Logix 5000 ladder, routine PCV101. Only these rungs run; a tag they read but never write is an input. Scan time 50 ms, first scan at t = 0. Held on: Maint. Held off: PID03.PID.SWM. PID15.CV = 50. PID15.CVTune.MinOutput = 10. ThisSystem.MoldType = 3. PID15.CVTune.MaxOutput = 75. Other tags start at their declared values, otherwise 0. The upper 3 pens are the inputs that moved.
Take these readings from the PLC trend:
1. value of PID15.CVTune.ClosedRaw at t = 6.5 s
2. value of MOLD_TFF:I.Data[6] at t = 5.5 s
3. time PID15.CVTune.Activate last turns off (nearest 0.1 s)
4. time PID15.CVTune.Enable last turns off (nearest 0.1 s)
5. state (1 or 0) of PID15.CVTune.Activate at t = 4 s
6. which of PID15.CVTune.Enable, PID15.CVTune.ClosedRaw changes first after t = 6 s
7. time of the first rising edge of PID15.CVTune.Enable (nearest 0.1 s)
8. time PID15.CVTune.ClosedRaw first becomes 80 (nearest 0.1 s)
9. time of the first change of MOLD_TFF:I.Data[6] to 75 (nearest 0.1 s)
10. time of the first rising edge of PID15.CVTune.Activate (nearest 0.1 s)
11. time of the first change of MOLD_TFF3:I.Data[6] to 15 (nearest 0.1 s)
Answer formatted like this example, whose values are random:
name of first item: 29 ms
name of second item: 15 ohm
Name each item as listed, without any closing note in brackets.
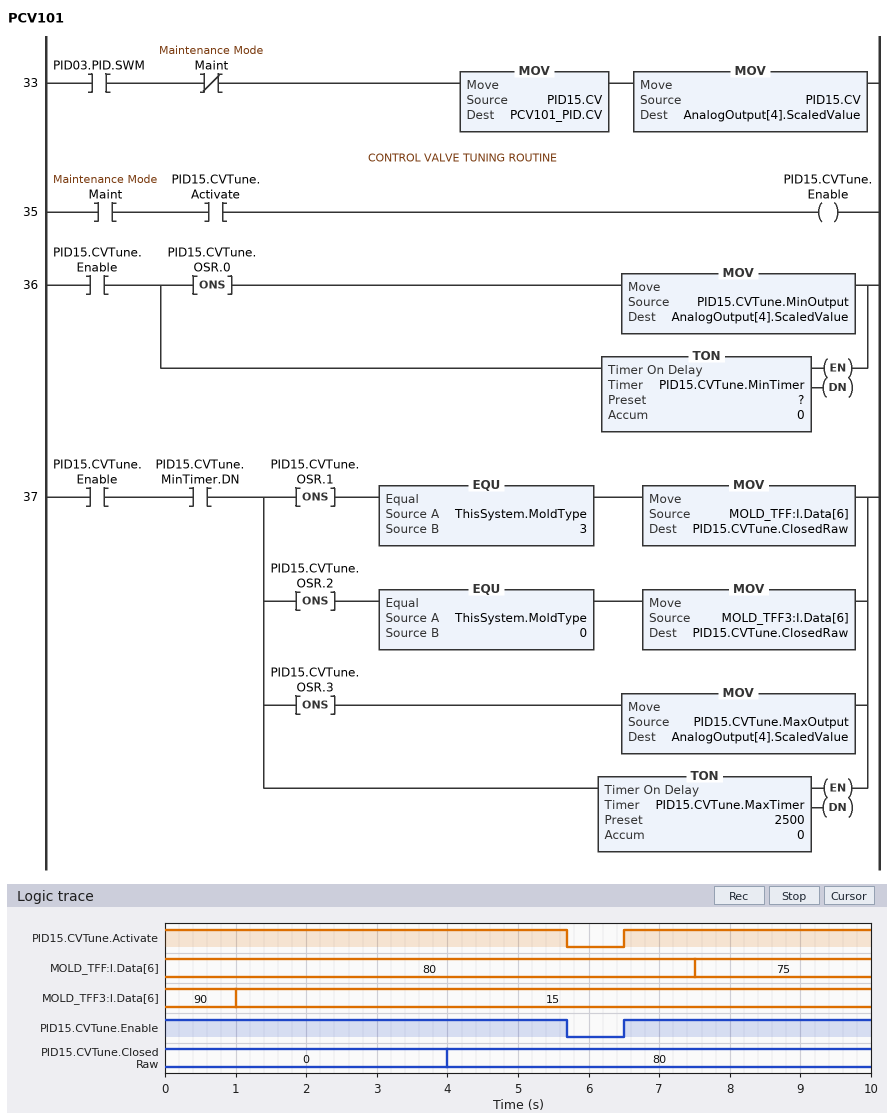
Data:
value of PID15.CVTune.ClosedRaw at t = 6.5 s: 80
value of MOLD_TFF:I.Data[6] at t = 5.5 s: 80
time PID15.CVTune.Activate last turns off: 5.7 s
time PID15.CVTune.Enable last turns off: 5.7 s
state (1 or 0) of PID15.CVTune.Activate at t = 4 s: 1
which of PID15.CVTune.Enable, PID15.CVTune.ClosedRaw changes first after t = 6 s: PID15.CVTune.Enable
time of the first rising edge of PID15.CVTune.Enable: 6.5 s
time PID15.CVTune.ClosedRaw first becomes 80: 4.0 s
time of the first change of MOLD_TFF:I.Data[6] to 75: 7.5 s
time of the first rising edge of PID15.CVTune.Activate: 6.5 s
time of the first change of MOLD_TFF3:I.Data[6] to 15: 1.0 s
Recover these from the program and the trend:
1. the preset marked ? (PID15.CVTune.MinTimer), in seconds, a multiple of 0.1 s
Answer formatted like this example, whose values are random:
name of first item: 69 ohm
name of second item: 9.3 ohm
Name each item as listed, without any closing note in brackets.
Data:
the preset marked ? (PID15.CVTune.MinTimer), in seconds, a multiple of 0.1 s: 4.0 s
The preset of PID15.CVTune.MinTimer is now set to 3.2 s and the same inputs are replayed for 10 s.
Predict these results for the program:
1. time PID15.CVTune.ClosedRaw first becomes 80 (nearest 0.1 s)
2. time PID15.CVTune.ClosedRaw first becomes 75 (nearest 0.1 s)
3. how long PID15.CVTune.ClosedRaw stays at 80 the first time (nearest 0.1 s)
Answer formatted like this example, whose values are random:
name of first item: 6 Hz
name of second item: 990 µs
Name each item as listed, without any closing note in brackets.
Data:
time PID15.CVTune.ClosedRaw first becomes 80: 3.2 s
time PID15.CVTune.ClosedRaw first becomes 75: 9.7 s
how long PID15.CVTune.ClosedRaw stays at 80 the first time: 6.5 s
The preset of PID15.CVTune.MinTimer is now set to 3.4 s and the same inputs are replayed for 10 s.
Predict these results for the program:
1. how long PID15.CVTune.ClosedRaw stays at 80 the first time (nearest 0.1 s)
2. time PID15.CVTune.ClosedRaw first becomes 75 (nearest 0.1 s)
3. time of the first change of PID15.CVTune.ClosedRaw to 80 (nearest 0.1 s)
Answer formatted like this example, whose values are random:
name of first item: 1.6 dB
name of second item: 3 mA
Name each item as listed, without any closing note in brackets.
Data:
how long PID15.CVTune.ClosedRaw stays at 80 the first time: 6.5 s
time PID15.CVTune.ClosedRaw first becomes 75: 9.9 s
time of the first change of PID15.CVTune.ClosedRaw to 80: 3.4 s
